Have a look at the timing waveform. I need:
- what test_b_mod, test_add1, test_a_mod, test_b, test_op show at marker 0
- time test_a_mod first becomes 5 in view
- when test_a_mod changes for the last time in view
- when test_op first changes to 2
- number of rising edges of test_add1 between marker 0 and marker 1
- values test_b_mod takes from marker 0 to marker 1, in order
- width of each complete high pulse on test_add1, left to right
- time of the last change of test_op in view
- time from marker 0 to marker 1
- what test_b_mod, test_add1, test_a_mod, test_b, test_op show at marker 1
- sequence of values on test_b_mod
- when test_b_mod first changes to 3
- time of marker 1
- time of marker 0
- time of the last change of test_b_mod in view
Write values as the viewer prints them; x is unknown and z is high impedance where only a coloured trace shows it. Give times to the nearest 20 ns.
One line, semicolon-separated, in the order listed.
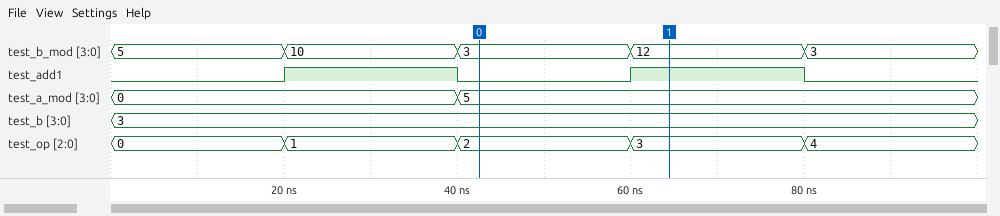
test_b_mod=3, test_add1=0, test_a_mod=5, test_b=3, test_op=2; 40 ns; 40 ns; 40 ns; 1; 3, 12; 20 ns, 20 ns; 80 ns; 20 ns; test_b_mod=12, test_add1=1, test_a_mod=5, test_b=3, test_op=3; 5, 10, 3, 12, 3; 40 ns; 60 ns; 40 ns; 80 ns
